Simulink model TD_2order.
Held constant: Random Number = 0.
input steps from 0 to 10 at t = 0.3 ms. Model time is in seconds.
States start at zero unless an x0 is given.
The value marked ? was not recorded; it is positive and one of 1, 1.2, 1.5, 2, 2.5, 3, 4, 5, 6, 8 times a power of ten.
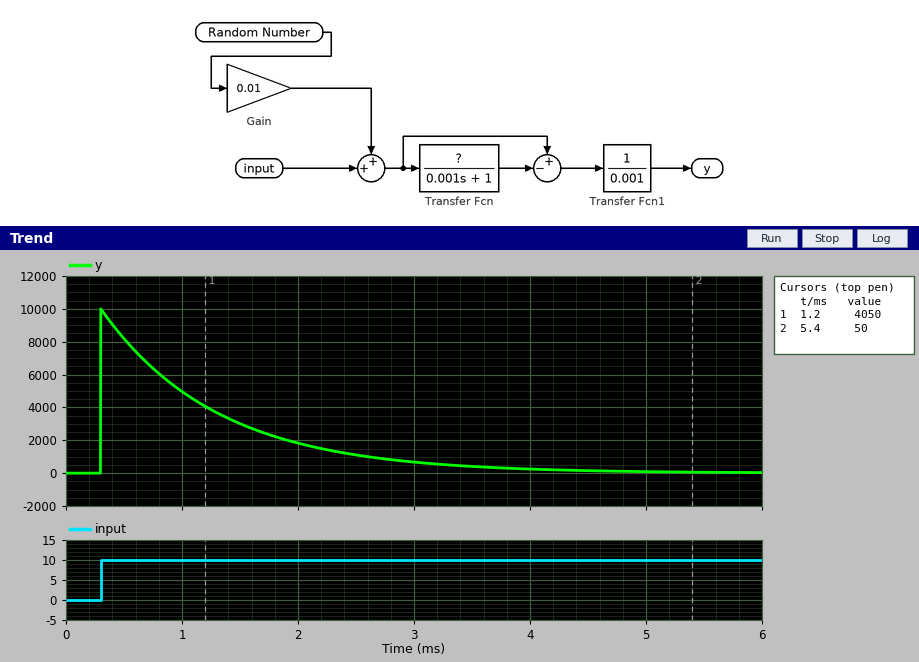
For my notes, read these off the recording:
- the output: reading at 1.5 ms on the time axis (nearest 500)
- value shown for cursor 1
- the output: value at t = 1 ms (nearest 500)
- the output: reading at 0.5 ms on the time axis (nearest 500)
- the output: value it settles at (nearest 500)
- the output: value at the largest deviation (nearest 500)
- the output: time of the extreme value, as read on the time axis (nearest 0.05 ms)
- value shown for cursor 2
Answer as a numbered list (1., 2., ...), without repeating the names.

1. 3000
2. 4050
3. 5000
4. 8000
5. 0
6. 10000
7. 0.30 ms
8. 50
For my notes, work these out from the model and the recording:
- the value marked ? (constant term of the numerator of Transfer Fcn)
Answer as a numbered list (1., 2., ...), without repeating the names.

1. 1
